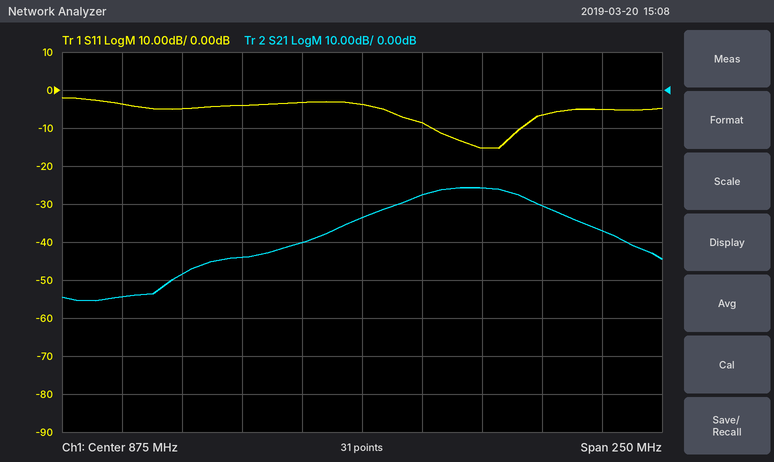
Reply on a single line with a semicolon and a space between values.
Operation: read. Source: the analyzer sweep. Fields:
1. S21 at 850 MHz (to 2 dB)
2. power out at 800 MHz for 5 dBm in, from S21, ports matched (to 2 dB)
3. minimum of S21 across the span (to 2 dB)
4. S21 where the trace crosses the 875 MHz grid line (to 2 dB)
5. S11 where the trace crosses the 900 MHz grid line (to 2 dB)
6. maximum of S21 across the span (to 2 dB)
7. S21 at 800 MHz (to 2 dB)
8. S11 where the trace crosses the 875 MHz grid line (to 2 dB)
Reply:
-40 dB; -44 dBm; -56 dB; -34 dB; -8 dB; -26 dB; -48 dB; -4 dB
